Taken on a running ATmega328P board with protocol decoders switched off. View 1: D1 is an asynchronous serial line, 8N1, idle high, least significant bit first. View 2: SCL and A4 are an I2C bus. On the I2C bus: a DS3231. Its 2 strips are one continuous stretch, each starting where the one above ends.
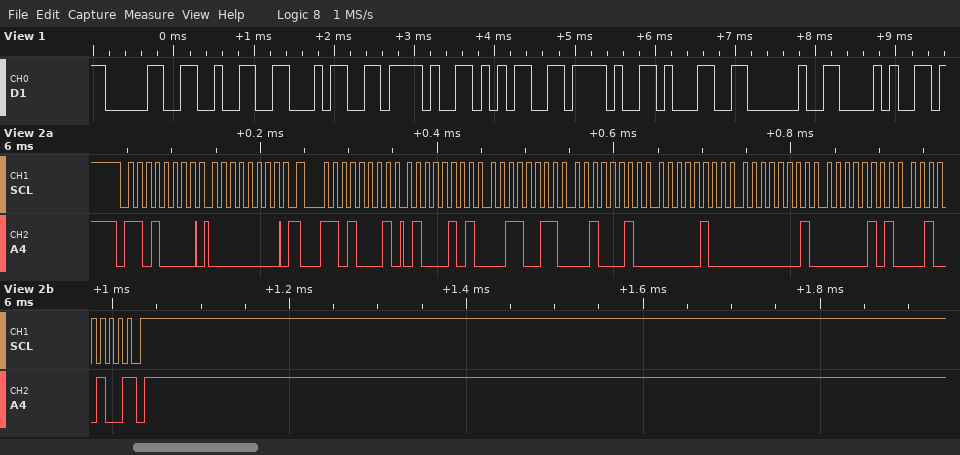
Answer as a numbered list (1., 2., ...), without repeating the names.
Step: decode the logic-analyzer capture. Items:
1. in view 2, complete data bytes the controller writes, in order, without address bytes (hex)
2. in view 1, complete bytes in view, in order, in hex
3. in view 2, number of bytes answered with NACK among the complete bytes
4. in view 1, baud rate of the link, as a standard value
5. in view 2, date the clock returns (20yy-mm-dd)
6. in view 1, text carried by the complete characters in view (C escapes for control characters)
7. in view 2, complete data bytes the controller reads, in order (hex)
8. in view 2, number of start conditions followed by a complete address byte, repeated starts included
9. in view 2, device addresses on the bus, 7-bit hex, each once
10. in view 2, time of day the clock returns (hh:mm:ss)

1. 00
2. 30 32 34 2F 35 2F 31 20 28
3. 1
4. 9600 baud
5. 2024-05-01
6. "024/5/1 ("
7. 45 33 22 04 01 05 24
8. 2
9. 0x68
10. 22:33:45
